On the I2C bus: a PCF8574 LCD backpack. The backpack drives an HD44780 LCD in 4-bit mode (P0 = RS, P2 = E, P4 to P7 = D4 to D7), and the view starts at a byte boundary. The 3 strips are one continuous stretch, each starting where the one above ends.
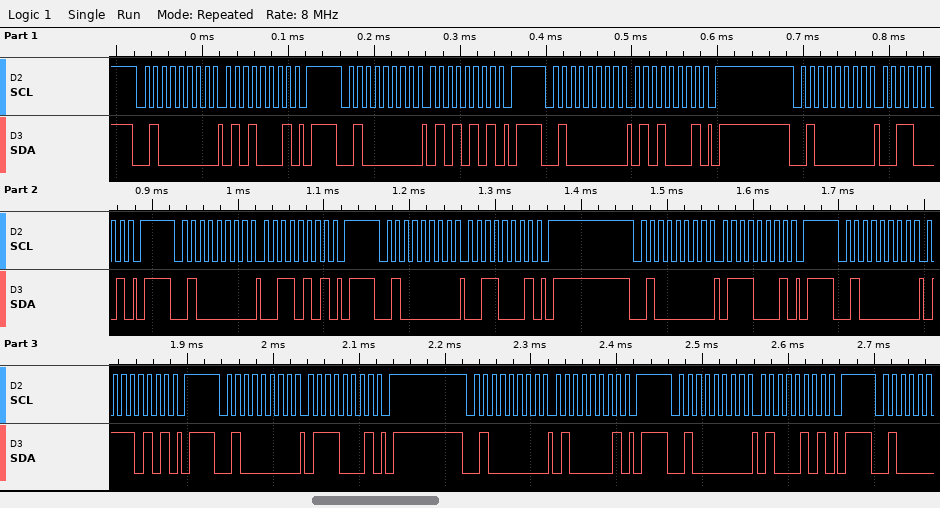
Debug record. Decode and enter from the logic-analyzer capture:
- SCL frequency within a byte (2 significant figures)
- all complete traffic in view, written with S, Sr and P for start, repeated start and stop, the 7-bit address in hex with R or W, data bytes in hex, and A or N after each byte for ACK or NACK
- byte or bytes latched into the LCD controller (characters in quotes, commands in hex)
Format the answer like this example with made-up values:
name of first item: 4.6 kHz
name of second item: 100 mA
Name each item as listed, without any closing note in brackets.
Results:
SCL frequency within a byte: 100 kHz
all complete traffic in view, written with S, Sr and P for start, repeated start and stop, the 7-bit address in hex with R or W, data bytes in hex, and A or N after each byte for ACK or NACK: S 20W A 51 A P S 20W A 55 A P S 20W A 51 A P S 20W A 31 A P S 20W A 35 A P S 20W A 31 A P S 20W A 71 A P S 20W A 75 A P S 20W A 71 A P S 20W A 41 A P S 20W A 45 A P
byte or bytes latched into the LCD controller: 'S'
